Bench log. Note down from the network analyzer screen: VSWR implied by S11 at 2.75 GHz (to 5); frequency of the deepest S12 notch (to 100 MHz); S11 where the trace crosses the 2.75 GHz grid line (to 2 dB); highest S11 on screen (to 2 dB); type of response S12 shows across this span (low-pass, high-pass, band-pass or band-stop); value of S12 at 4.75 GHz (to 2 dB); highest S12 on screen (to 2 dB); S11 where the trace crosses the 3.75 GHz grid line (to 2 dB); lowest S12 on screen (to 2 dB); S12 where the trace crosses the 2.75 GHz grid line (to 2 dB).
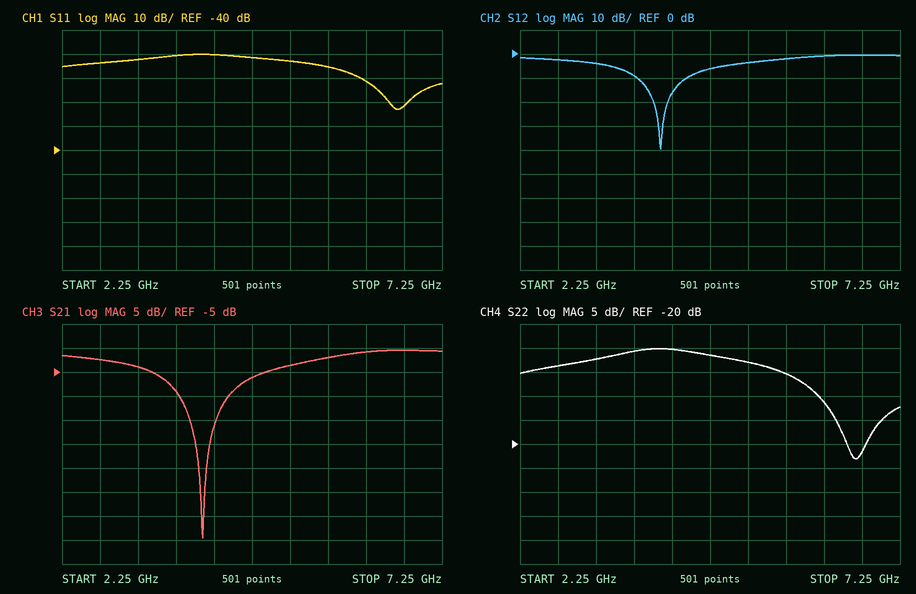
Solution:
5
4.1 GHz
-4 dB
0 dB
band-stop
-6 dB
0 dB
0 dB
-40 dB
-2 dB
